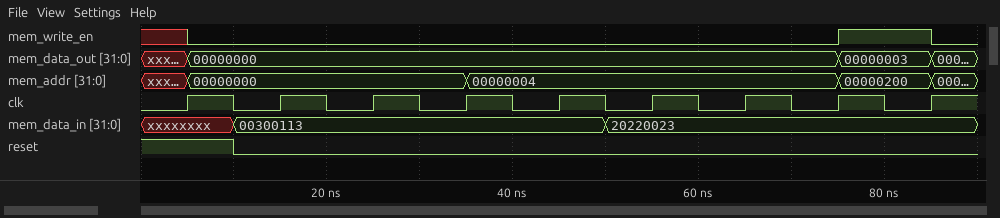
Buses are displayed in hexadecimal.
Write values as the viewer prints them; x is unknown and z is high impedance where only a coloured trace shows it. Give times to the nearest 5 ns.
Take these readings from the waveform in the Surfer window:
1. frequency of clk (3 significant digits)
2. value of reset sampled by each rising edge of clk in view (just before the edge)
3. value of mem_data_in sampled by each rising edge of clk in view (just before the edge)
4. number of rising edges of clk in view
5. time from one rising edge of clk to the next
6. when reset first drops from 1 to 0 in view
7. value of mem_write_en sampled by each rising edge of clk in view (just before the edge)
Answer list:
100 MHz
1 0 0 0 0 0 0 0 0
xxxxxxxx, 00300113, 00300113, 00300113, 00300113, 20220023, 20220023, 20220023, 20220023
9
10 ns
10 ns
x 0 0 0 0 0 0 0 1
